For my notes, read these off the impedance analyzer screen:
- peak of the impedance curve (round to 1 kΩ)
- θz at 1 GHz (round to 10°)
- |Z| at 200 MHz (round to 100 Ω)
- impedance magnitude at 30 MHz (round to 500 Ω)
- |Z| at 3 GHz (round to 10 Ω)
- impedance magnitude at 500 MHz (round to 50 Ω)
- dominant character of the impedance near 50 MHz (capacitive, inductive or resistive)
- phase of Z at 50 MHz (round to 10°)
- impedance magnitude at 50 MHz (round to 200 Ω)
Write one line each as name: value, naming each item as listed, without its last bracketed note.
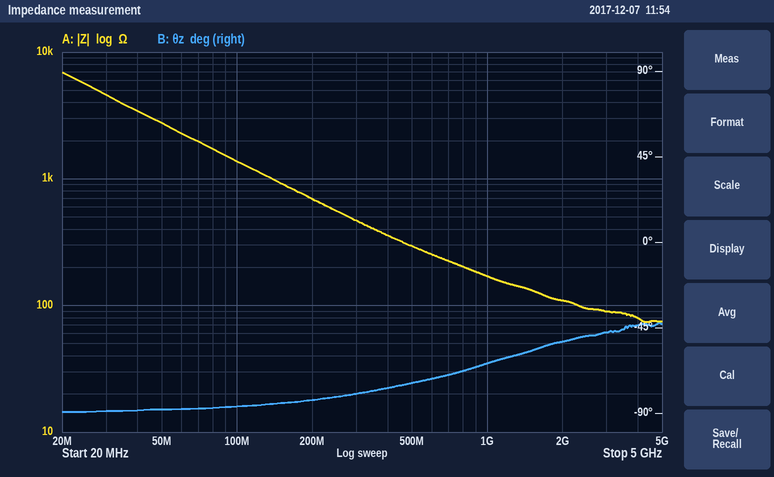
peak of the impedance curve: 7 kΩ
θz at 1 GHz: -60°
|Z| at 200 MHz: 700 Ω
impedance magnitude at 30 MHz: 4.5 kΩ
|Z| at 3 GHz: 90 Ω
impedance magnitude at 500 MHz: 300 Ω
dominant character of the impedance near 50 MHz: capacitive
phase of Z at 50 MHz: -90°
impedance magnitude at 50 MHz: 2.8 kΩ
